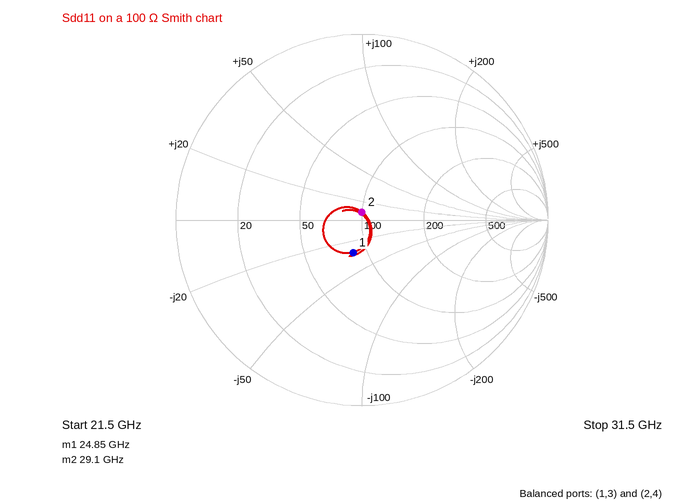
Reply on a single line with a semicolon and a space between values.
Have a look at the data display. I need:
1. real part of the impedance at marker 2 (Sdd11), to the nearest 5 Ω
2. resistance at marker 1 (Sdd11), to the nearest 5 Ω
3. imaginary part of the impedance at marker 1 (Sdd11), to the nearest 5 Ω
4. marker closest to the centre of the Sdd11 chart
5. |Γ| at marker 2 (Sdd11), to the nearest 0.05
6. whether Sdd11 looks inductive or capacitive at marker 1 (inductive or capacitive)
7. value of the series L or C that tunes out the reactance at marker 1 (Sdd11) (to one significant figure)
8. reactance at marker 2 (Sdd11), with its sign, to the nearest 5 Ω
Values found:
100 Ω; 85 Ω; -30 Ω; marker 2; 0.05; capacitive; 200 pH; +10 Ω
